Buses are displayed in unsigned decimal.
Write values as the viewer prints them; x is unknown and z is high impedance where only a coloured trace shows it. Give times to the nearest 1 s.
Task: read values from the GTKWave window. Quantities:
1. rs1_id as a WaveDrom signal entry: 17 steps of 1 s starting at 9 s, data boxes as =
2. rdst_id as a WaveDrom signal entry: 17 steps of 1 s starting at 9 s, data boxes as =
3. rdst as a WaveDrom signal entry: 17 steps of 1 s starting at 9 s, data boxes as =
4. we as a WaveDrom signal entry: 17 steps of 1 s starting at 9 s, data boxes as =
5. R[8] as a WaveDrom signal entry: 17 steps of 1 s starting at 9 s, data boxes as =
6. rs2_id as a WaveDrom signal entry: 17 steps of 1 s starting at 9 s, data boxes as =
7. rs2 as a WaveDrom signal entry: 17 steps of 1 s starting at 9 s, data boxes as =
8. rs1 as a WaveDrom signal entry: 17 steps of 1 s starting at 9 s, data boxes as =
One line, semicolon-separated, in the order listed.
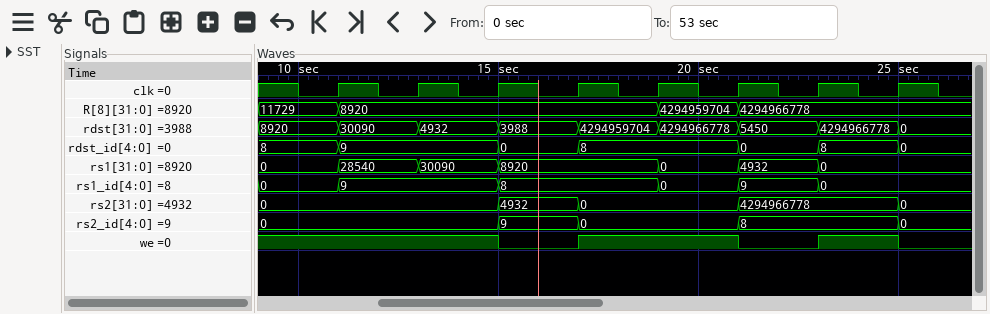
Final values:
{name: 'rs1_id', wave: '=.=...=...=.=.=..', data: '0 9 8 0 9 0'}; {name: 'rdst_id', wave: '=.=...=.=...=.=.=', data: '8 9 0 8 0 8 0'}; {name: 'rdst', wave: '=.=.=.=.=.=.=.=.=', data: '8920 30090 4932 3988 4294959704 4294966778 5450 4294966778 0'}; {name: 'we', wave: '1.....0.1...0.1.0'}; {name: 'R[8]', wave: '=.=.......=.=....', data: '11729 8920 4294959704 4294966778'}; {name: 'rs2_id', wave: '=.....=.=...=...=', data: '0 9 0 8 0'}; {name: 'rs2', wave: '=.....=.=...=...=', data: '0 4932 0 4294966778 0'}; {name: 'rs1', wave: '=.=.=.=...=.=.=..', data: '0 28540 30090 8920 0 4932 0'}
